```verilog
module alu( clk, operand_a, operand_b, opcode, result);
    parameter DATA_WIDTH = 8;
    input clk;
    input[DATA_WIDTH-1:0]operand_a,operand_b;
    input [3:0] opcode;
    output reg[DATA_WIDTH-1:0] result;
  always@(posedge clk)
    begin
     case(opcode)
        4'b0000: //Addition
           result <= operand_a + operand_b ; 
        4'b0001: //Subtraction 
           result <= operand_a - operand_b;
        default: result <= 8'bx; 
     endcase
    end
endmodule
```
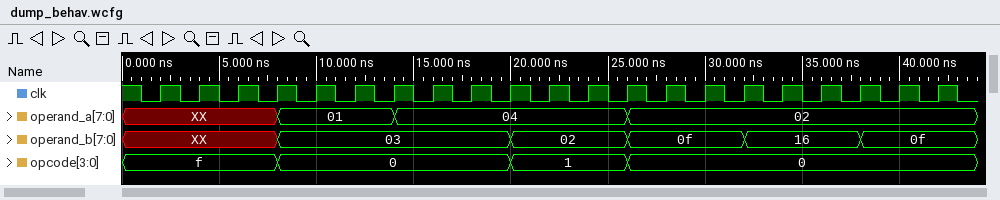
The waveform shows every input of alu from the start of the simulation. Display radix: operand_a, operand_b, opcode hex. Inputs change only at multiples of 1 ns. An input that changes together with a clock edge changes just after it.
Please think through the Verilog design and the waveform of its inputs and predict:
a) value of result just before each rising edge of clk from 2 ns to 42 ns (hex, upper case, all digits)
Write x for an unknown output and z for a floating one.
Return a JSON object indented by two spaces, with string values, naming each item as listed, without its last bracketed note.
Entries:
{
  "value of result just before each rising edge of clk from 2 ns to 42 ns": "x, x, x, x, x, 04, 04, 04, 07, 07, 07, 02, 02, 02, 11, 11, 11, 18, 18, 18, 11"
}
